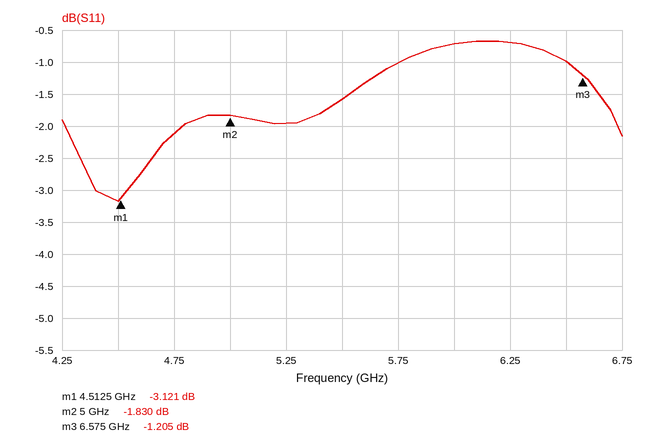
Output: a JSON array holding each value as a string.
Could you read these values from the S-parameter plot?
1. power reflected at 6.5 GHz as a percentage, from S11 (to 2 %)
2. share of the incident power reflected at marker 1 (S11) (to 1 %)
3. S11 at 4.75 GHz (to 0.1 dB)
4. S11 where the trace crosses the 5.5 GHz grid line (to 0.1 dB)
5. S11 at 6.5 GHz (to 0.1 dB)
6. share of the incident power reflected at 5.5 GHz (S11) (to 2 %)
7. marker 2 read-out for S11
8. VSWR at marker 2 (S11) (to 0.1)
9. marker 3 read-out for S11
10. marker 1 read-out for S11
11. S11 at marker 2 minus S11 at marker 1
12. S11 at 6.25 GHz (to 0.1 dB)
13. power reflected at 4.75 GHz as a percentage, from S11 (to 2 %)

["80 %", "49 %", "-2.1 dB", "-1.6 dB", "-1.0 dB", "70 %", "-1.830 dB", "9.5", "-1.205 dB", "-3.121 dB", "1.291 dB", "-0.7 dB", "62 %"]
